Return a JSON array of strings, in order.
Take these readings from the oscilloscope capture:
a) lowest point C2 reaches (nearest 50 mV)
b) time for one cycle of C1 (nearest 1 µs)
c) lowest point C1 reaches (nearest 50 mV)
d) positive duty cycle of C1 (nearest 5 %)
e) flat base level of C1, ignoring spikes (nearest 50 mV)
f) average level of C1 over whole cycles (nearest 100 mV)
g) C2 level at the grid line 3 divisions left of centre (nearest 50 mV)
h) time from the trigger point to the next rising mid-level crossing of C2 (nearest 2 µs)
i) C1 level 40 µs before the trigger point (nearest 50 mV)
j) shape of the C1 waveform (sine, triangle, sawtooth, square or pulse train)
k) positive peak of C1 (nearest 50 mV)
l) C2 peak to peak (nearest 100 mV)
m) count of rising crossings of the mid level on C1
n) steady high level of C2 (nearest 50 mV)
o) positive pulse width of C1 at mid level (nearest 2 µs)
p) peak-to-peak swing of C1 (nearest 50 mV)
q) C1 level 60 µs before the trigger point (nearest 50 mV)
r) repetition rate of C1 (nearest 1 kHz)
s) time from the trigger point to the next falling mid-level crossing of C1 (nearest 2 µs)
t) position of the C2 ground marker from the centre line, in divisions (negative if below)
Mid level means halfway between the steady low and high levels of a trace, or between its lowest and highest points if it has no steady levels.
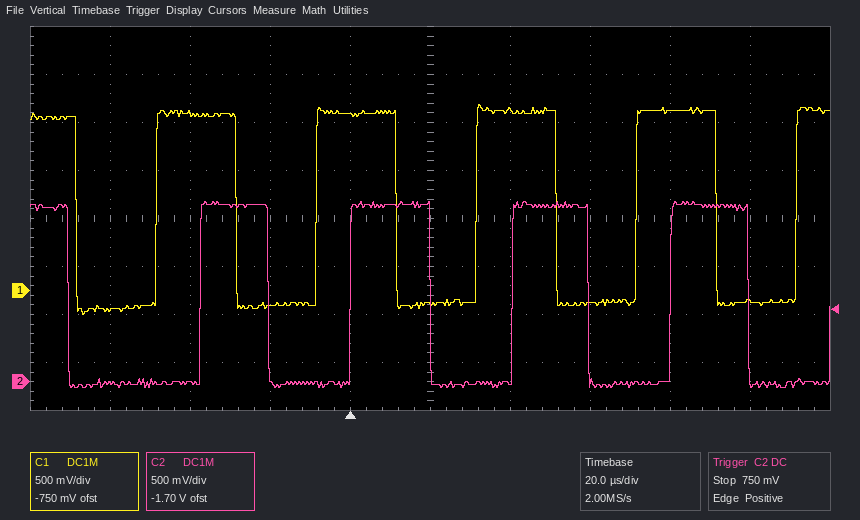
["-50 mV", "40 µs", "-250 mV", "50 %", "-150 mV", "900 mV", "0 mV", "40 µs", "1.85 V", "square", "1.95 V", "1.90 V", "5", "1.85 V", "20 µs", "2.20 V", "-200 mV", "25 kHz", "12 µs", "-3.4 div"]
